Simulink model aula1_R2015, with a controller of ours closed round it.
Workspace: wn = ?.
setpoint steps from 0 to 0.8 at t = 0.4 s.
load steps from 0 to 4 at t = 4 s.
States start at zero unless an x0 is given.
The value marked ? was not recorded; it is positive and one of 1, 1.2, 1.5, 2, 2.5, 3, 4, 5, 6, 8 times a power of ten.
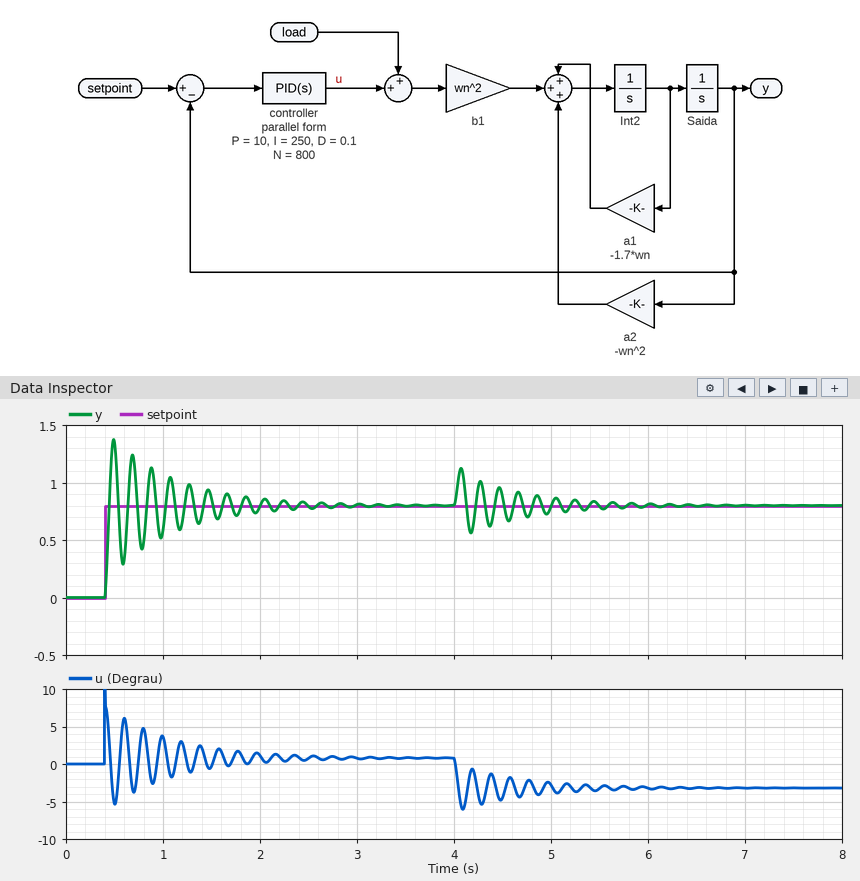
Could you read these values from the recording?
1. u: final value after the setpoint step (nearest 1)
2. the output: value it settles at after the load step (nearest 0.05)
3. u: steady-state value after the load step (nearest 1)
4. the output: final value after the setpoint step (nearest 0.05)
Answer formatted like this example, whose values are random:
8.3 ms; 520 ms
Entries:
1; 0.80; -3; 0.80
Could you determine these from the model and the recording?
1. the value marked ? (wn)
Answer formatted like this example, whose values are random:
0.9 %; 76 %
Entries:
10
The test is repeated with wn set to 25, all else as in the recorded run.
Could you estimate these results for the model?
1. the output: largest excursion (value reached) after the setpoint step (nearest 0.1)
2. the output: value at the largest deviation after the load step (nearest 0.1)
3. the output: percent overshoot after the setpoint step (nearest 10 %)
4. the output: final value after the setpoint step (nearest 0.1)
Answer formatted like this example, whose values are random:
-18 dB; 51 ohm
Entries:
1.0; 1.1; 20 %; 0.8
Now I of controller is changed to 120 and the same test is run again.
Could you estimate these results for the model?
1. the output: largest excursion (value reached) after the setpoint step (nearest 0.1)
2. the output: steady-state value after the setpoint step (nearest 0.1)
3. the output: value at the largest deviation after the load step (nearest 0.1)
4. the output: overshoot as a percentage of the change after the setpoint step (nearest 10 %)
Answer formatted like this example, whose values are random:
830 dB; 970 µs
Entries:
1.2; 0.8; 1.2; 50 %
